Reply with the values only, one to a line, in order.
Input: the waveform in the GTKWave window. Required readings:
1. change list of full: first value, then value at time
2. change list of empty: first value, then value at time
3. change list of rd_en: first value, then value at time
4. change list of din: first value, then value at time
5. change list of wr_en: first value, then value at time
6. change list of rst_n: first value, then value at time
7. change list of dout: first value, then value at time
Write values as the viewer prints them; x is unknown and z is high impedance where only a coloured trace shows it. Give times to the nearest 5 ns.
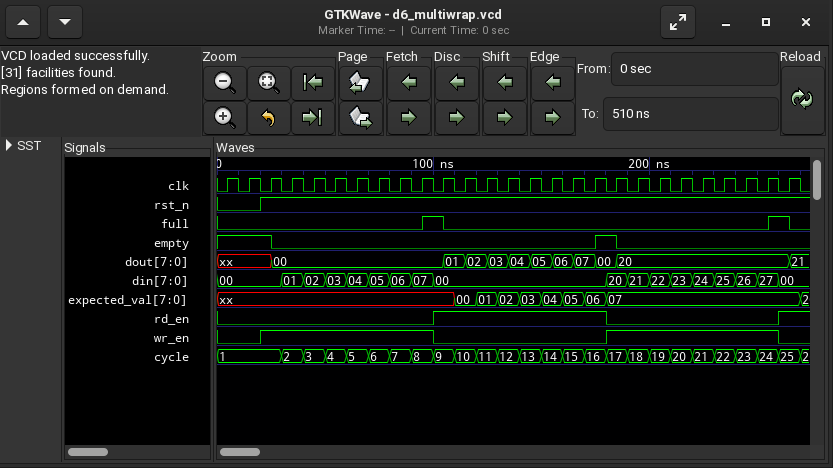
0, 1 at 95 ns, 0 at 105 ns, 1 at 255 ns, 0 at 265 ns
1, 0 at 25 ns, 1 at 175 ns, 0 at 185 ns
0, 1 at 100 ns, 0 at 180 ns, 1 at 260 ns
00, 01 at 30 ns, 02 at 40 ns, 03 at 50 ns, 04 at 60 ns, 05 at 70 ns, 06 at 80 ns, 07 at 90 ns, 00 at 100 ns, 20 at 180 ns, 21 at 190 ns, 22 at 200 ns, 23 at 210 ns, 24 at 220 ns, 25 at 230 ns, 26 at 240 ns, 27 at 250 ns, 00 at 260 ns
0, 1 at 20 ns, 0 at 100 ns, 1 at 180 ns, 0 at 260 ns
0, 1 at 20 ns
xx, 00 at 25 ns, 01 at 105 ns, 02 at 115 ns, 03 at 125 ns, 04 at 135 ns, 05 at 145 ns, 06 at 155 ns, 07 at 165 ns, 00 at 175 ns, 20 at 185 ns, 21 at 265 ns
